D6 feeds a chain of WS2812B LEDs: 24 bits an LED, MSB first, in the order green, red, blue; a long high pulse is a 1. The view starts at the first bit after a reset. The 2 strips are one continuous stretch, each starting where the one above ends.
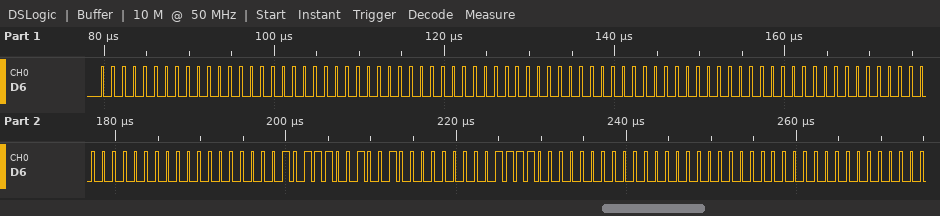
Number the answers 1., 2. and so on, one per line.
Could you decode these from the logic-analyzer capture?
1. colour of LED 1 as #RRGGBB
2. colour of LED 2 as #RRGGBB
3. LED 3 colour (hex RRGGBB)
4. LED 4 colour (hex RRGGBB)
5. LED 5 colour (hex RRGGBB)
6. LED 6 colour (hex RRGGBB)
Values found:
1. #000000
2. #000000
3. #000000
4. #000000
5. #20B90F
6. #000000
